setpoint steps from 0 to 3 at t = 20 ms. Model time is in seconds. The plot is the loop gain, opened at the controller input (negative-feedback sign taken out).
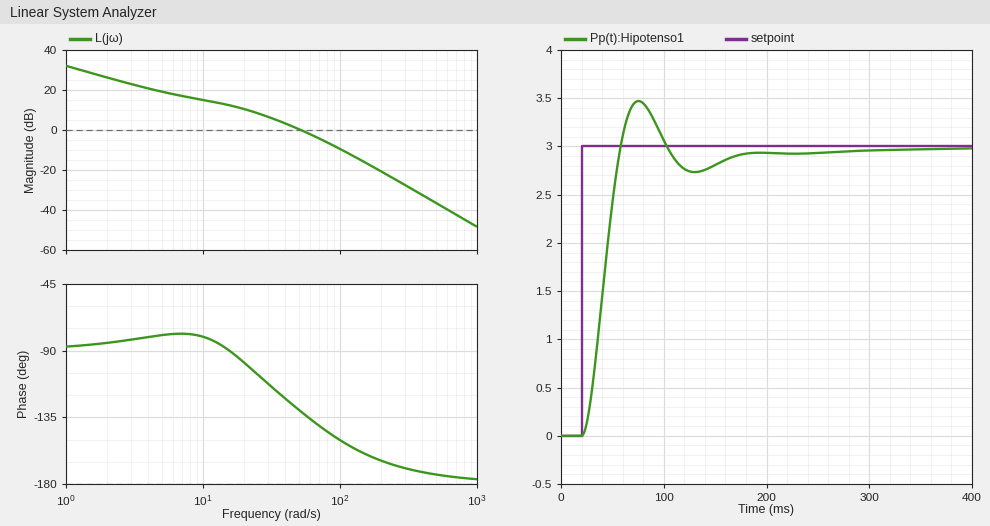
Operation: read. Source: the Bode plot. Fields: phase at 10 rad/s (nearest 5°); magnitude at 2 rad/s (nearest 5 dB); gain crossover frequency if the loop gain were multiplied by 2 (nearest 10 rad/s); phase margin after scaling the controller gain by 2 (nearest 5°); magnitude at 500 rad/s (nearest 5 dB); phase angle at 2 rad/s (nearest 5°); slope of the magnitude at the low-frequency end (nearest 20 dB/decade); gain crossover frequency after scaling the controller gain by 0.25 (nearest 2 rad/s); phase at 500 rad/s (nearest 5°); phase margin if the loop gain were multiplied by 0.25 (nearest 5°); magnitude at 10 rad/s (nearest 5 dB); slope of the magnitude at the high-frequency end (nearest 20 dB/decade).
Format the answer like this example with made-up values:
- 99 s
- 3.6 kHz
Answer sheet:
- -80°
- 25 dB
- 80 rad/s
- 35°
- -35 dB
- -85°
- -20 dB/decade
- 16 rad/s
- -175°
- 90°
- 15 dB
- -40 dB/decade
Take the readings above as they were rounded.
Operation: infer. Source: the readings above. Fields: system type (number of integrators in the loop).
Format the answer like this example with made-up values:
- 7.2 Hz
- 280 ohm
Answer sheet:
- 1
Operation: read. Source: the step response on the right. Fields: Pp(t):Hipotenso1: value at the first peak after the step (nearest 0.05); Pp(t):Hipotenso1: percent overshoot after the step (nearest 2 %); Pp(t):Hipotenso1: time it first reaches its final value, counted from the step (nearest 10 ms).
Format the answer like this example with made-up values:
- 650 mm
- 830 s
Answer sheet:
- 3.45
- 16 %
- 40 ms
